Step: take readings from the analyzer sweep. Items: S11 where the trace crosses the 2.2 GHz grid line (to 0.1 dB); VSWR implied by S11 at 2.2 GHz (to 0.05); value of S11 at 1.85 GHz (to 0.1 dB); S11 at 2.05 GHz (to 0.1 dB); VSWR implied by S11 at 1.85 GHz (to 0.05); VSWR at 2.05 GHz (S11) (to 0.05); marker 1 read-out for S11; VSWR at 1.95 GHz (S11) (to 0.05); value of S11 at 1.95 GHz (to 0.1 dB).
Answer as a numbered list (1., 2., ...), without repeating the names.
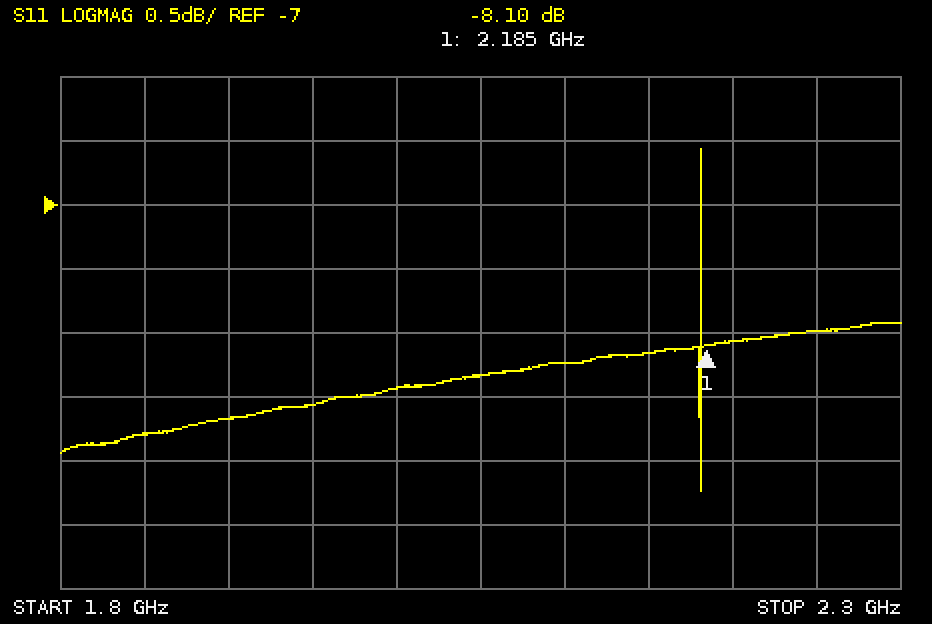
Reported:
1. -8.1 dB
2. 2.30
3. -8.8 dB
4. -8.3 dB
5. 2.15
6. 2.25
7. -8.10 dB
8. 2.20
9. -8.6 dB
